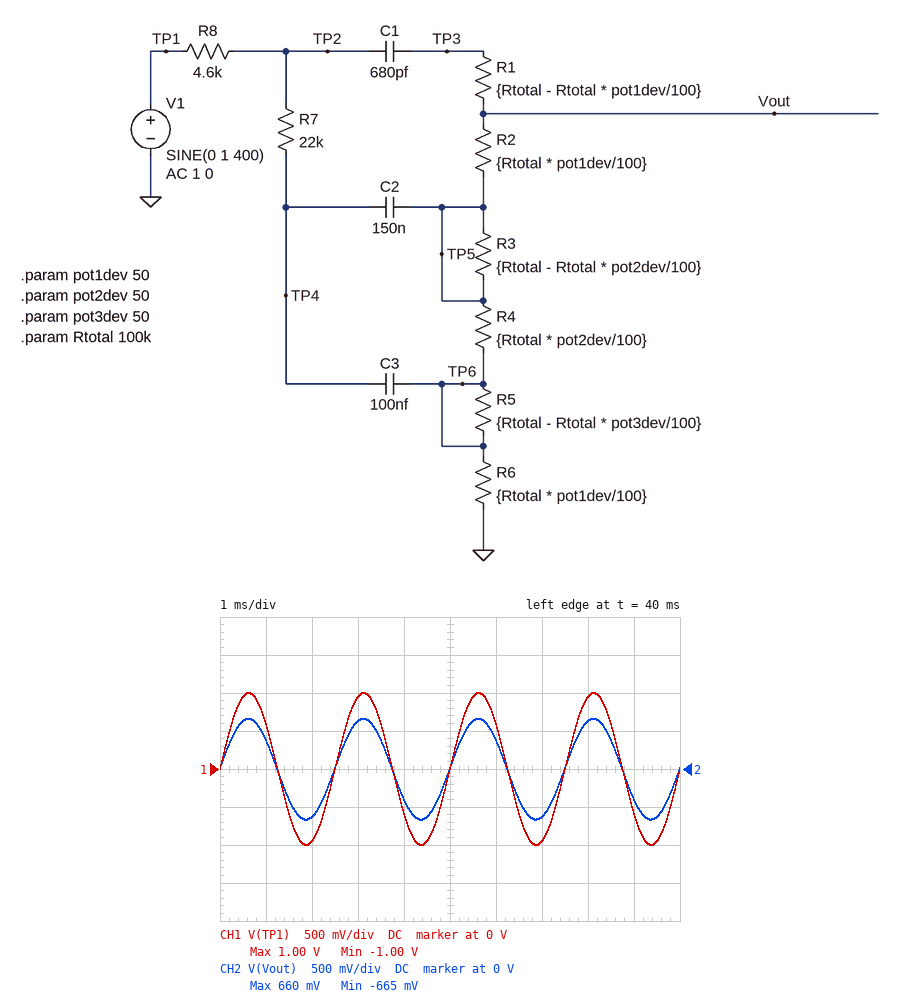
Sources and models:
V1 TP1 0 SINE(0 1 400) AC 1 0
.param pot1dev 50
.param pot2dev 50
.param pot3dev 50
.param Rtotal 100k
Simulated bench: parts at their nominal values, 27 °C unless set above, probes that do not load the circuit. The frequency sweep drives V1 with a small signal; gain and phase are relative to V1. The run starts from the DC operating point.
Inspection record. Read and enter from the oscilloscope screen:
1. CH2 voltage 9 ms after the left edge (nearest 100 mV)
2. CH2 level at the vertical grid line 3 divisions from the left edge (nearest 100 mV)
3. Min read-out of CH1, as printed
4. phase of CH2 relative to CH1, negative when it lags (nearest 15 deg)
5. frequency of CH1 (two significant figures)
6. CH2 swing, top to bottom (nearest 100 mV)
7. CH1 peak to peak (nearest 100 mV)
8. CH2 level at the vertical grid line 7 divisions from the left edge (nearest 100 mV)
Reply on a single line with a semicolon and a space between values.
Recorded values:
-400 mV; 600 mV; -1.00 V; 0 deg; 400 Hz; 1.3 V; 2.0 V; -600 mV
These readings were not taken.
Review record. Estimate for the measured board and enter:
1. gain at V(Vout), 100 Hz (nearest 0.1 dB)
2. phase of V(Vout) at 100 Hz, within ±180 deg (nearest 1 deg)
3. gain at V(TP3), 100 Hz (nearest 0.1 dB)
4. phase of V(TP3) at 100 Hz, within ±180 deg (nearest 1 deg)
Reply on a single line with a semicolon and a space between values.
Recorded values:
-3.0 dB; -2 deg; -3.0 dB; -2 deg
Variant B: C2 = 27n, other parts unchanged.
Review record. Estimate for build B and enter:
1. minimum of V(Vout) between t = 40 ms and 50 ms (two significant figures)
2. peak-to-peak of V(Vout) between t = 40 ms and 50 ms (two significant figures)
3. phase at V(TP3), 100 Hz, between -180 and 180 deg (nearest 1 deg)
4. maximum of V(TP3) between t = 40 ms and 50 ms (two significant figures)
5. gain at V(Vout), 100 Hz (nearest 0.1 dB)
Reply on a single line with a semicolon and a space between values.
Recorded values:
-680 mV; 1.4 V; 6 deg; 680 mV; -2.7 dB
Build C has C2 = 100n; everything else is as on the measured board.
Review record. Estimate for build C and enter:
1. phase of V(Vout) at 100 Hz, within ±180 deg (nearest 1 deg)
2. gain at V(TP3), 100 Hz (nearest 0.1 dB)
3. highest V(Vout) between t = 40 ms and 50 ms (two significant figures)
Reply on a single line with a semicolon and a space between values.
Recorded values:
-1 deg; -2.9 dB; 660 mV
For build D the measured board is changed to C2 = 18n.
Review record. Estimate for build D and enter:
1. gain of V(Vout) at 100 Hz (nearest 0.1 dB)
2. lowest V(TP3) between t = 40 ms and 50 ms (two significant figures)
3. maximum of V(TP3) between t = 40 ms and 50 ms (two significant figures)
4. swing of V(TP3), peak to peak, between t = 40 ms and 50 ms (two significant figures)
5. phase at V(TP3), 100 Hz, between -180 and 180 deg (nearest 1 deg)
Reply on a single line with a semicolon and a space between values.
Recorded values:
-2.8 dB; -690 mV; 690 mV; 1.4 V; 8 deg
